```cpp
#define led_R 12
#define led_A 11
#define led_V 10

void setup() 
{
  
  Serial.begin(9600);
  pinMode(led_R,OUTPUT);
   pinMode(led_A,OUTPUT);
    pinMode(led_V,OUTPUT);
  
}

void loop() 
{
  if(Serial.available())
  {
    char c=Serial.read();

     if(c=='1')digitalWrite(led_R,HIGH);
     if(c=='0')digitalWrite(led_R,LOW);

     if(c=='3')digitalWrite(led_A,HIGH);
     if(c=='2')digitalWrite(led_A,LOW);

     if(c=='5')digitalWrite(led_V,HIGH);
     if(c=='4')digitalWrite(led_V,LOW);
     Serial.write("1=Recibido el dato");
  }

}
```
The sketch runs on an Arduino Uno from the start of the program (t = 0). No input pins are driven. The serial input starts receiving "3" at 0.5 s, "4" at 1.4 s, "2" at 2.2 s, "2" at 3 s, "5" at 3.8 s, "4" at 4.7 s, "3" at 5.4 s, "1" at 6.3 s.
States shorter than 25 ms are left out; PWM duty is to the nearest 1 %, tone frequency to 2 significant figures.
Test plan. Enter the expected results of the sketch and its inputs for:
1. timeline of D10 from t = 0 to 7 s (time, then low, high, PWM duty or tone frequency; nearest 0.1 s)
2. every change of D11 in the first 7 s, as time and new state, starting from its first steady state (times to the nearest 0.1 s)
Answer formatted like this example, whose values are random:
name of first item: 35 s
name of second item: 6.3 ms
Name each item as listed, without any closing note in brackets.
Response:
timeline of D10 from t = 0 to 7 s: 0 s low; 3.8 s high; 4.7 s low
every change of D11 in the first 7 s, as time and new state, starting from its first steady state: 0 s low; 0.5 s high; 2.2 s low; 5.4 s high
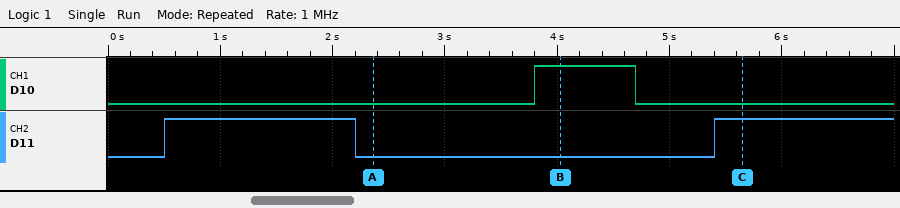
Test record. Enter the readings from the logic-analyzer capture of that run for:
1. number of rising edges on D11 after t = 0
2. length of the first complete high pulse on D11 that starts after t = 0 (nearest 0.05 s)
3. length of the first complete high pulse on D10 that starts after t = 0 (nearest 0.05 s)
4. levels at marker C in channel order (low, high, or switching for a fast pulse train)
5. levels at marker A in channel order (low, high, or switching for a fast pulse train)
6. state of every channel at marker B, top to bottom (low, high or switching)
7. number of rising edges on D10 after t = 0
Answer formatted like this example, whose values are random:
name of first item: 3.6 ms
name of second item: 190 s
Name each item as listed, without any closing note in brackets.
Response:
number of rising edges on D11 after t = 0: 2
length of the first complete high pulse on D11 that starts after t = 0: 1.70 s
length of the first complete high pulse on D10 that starts after t = 0: 0.90 s
levels at marker C in channel order: D10 low, D11 high
levels at marker A in channel order: D10 low, D11 low
state of every channel at marker B, top to bottom: D10 high, D11 low
number of rising edges on D10 after t = 0: 1
